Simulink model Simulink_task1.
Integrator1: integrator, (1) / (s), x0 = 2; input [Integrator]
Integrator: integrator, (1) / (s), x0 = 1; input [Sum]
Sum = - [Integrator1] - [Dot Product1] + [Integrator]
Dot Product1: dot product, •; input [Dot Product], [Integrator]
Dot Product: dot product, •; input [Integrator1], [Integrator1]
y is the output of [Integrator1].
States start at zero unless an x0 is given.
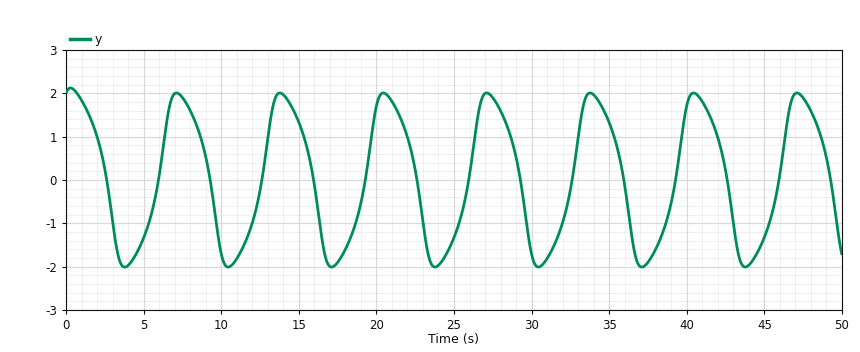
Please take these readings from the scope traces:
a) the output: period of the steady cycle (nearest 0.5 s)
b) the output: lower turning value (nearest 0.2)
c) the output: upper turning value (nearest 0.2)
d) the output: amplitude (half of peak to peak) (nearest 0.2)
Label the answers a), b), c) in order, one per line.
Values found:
a) 6.5 s
b) -2.0
c) 2.0
d) 2.0
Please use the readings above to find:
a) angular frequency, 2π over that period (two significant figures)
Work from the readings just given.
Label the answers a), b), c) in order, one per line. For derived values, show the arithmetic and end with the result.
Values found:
a) 2π / 6.5 = 0.97 rad/s
